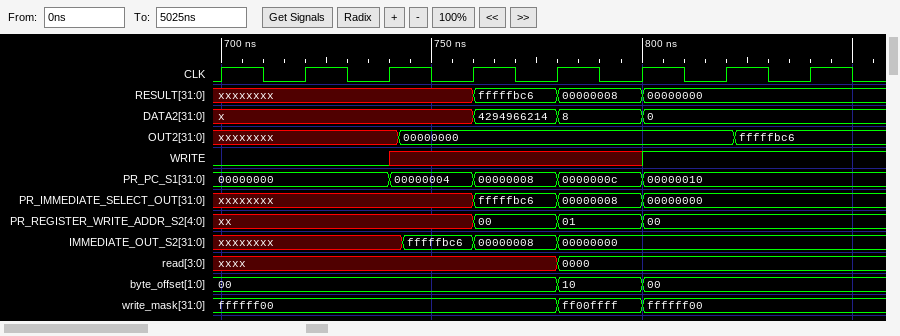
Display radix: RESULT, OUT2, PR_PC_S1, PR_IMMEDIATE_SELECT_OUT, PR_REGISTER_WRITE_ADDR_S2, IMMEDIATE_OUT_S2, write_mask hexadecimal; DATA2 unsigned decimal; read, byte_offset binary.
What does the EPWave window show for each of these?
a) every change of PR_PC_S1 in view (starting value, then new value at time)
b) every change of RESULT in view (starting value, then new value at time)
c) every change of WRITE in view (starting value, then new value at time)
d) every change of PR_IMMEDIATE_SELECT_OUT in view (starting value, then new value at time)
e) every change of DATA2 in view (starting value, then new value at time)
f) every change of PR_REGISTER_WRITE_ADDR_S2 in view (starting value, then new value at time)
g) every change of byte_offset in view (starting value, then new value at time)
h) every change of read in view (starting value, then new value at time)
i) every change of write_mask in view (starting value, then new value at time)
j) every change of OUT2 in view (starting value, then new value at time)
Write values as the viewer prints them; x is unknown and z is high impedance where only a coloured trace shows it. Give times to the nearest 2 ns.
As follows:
00000000, 00000004 at 740 ns, 00000008 at 760 ns, 0000000c at 780 ns, 00000010 at 800 ns
xxxxxxxx, fffffbc6 at 760 ns, 00000008 at 780 ns, 00000000 at 800 ns
0, x at 740 ns, 1 at 800 ns
xxxxxxxx, fffffbc6 at 760 ns, 00000008 at 780 ns, 00000000 at 800 ns
x, 4294966214 at 760 ns, 8 at 780 ns, 0 at 800 ns
xx, 00 at 760 ns, 01 at 780 ns, 00 at 800 ns
00, 10 at 780 ns, 00 at 800 ns
xxxx, 0000 at 780 ns
ffffff00, ff00ffff at 780 ns, ffffff00 at 800 ns
xxxxxxxx, 00000000 at 742 ns, fffffbc6 at 822 ns
